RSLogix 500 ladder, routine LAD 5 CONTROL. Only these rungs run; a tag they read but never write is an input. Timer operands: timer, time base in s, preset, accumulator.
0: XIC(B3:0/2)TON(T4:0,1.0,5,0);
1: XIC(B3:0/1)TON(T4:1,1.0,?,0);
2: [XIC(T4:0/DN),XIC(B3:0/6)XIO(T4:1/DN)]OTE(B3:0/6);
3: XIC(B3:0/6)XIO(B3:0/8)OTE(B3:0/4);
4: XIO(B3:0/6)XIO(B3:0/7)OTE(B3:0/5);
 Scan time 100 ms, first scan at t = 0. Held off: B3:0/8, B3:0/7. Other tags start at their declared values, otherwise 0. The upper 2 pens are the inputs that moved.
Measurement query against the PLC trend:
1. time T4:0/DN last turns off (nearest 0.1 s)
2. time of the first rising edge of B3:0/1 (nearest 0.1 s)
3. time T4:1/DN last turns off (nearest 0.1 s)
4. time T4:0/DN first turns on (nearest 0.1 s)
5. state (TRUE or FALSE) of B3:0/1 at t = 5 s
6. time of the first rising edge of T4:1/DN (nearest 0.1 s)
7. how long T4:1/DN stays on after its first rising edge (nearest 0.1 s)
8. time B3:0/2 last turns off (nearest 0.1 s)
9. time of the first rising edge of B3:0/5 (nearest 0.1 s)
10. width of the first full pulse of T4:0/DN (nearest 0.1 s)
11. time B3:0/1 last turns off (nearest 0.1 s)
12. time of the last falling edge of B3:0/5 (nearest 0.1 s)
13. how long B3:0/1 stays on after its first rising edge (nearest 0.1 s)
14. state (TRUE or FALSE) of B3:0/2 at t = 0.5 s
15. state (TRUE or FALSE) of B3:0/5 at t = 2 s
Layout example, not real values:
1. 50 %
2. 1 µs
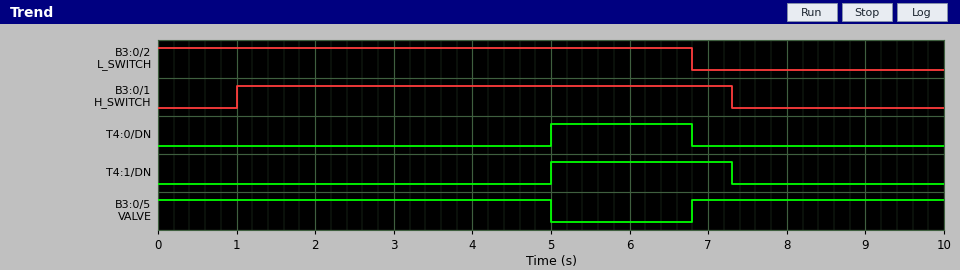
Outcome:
1. 6.8 s
2. 1.0 s
3. 7.3 s
4. 5.0 s
5. TRUE
6. 5.0 s
7. 2.3 s
8. 6.8 s
9. 6.8 s
10. 1.8 s
11. 7.3 s
12. 5.0 s
13. 6.3 s
14. TRUE
15. TRUE
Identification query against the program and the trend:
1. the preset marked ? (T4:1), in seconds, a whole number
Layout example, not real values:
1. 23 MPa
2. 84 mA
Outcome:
1. 4 s
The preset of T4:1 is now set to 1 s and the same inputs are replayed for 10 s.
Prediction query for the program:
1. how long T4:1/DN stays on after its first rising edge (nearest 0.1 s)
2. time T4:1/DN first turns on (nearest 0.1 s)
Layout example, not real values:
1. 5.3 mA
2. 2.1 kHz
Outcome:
1. 5.3 s
2. 2.0 s
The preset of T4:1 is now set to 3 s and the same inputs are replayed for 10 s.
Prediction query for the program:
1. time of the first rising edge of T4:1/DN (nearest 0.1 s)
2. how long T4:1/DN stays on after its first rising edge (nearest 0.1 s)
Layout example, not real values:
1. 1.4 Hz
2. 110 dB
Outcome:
1. 4.0 s
2. 3.3 s
